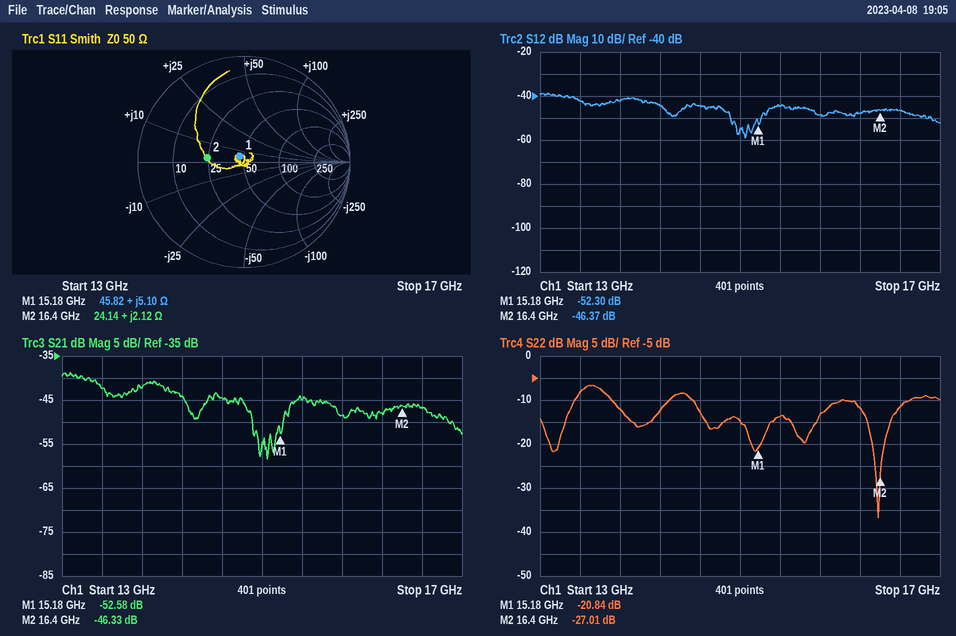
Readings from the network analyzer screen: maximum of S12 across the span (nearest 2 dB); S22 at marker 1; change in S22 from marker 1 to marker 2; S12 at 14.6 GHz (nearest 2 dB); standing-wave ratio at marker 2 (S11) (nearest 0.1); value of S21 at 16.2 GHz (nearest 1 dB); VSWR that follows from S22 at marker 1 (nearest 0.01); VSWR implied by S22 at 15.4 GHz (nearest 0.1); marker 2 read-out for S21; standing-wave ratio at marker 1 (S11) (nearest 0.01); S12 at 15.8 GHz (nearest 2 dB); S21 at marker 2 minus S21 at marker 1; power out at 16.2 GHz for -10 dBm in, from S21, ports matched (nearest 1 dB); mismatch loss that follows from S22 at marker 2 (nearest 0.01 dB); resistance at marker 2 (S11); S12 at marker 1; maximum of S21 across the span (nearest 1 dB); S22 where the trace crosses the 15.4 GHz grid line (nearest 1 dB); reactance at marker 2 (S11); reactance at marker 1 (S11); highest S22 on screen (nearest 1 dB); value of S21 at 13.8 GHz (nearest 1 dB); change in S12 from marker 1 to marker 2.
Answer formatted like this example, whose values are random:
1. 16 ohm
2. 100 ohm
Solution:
1. -38 dB
2. -20.84 dB
3. -6.17 dB
4. -44 dB
5. 2.1
6. -48 dB
7. 1.20
8. 1.5
9. -46.33 dB
10. 1.15
11. -48 dB
12. 6.25 dB
13. -58 dBm
14. 0.01 dB
15. 24.14 Ω
16. -52.30 dB
17. -39 dB
18. -14 dB
19. +2.12 Ω
20. +5.10 Ω
21. -7 dB
22. -42 dB
23. 5.93 dB
